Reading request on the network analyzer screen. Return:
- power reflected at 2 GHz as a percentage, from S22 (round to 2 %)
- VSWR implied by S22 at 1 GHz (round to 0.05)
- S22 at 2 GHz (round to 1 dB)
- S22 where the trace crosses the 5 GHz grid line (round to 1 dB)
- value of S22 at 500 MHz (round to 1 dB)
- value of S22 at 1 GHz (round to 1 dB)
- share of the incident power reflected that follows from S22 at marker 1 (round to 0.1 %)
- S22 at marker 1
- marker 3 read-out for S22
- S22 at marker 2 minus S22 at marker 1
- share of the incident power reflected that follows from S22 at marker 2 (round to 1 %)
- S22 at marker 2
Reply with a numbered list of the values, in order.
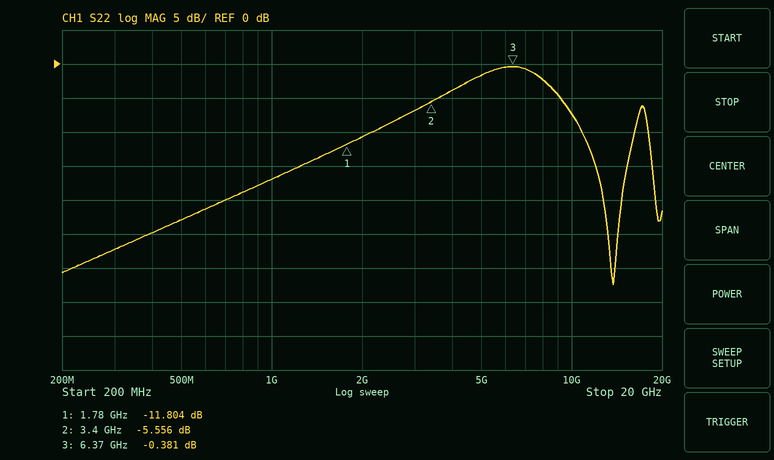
1. 8 %
2. 1.35
3. -11 dB
4. -2 dB
5. -23 dB
6. -17 dB
7. 6.6 %
8. -11.804 dB
9. -0.381 dB
10. 6.248 dB
11. 28 %
12. -5.556 dB
